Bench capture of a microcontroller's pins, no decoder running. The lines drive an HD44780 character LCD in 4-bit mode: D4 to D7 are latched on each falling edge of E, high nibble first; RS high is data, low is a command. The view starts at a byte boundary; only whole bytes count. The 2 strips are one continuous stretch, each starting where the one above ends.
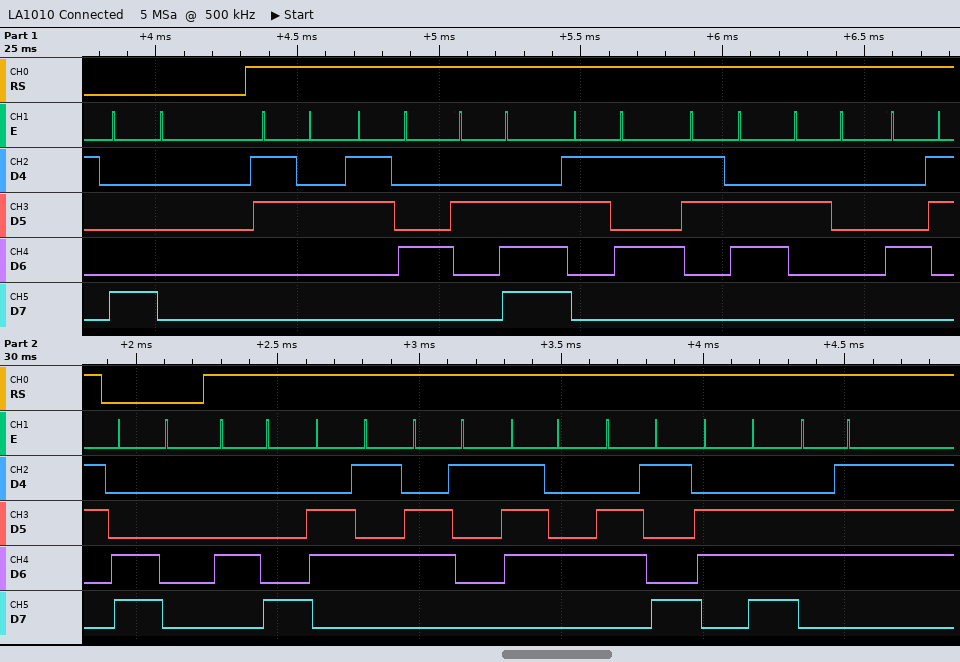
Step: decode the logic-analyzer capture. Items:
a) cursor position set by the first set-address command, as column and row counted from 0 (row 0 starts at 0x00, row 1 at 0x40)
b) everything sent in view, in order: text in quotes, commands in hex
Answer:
column 0, row 0
0x80 "24.56 C" 0xC0 "Heating"
